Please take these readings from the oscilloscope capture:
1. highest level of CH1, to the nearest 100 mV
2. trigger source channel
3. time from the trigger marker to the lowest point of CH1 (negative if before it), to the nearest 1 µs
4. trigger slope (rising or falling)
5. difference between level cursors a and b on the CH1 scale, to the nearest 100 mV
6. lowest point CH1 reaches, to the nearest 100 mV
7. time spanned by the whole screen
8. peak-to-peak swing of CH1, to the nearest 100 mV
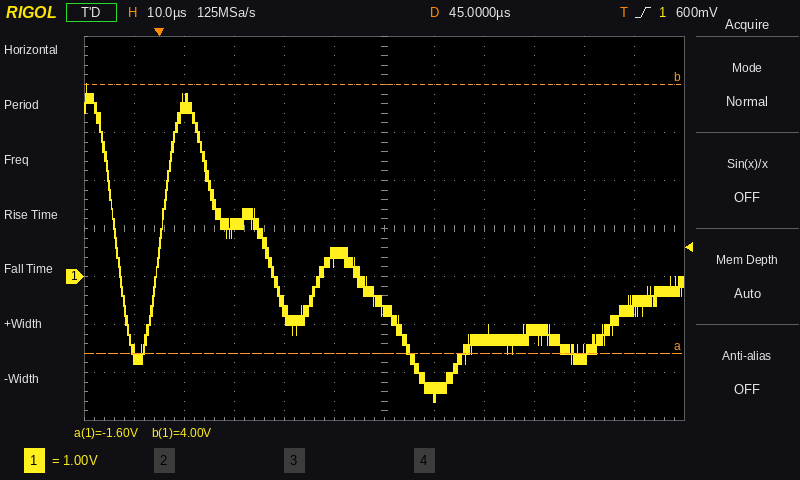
4.0 V
CH1
+55 µs
rising
5.6 V
-2.6 V
120 µs
6.6 V
